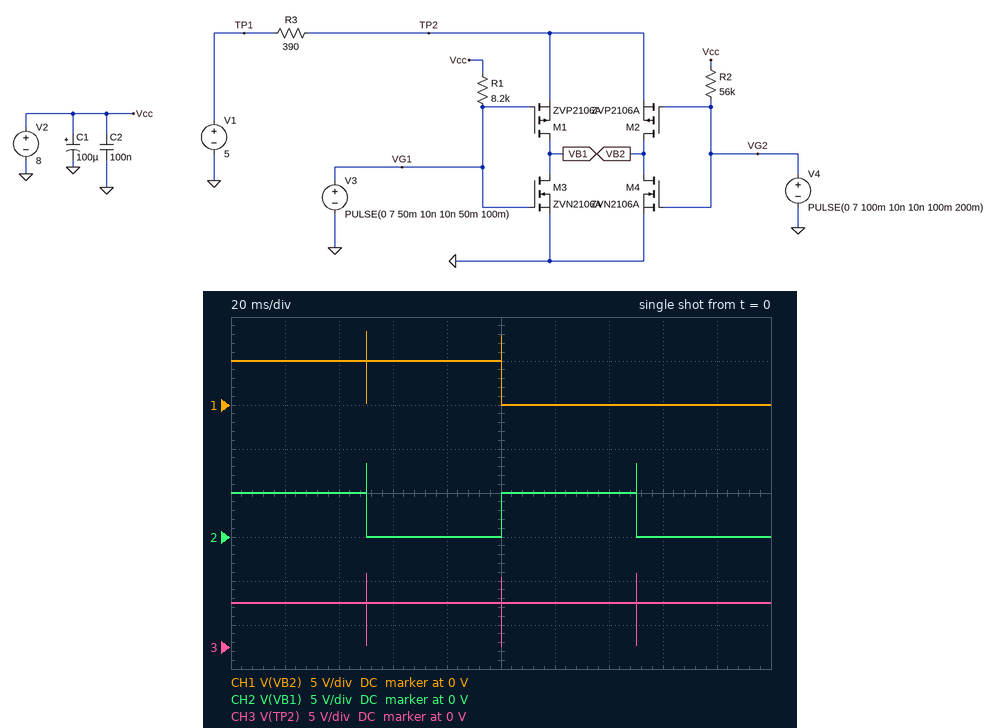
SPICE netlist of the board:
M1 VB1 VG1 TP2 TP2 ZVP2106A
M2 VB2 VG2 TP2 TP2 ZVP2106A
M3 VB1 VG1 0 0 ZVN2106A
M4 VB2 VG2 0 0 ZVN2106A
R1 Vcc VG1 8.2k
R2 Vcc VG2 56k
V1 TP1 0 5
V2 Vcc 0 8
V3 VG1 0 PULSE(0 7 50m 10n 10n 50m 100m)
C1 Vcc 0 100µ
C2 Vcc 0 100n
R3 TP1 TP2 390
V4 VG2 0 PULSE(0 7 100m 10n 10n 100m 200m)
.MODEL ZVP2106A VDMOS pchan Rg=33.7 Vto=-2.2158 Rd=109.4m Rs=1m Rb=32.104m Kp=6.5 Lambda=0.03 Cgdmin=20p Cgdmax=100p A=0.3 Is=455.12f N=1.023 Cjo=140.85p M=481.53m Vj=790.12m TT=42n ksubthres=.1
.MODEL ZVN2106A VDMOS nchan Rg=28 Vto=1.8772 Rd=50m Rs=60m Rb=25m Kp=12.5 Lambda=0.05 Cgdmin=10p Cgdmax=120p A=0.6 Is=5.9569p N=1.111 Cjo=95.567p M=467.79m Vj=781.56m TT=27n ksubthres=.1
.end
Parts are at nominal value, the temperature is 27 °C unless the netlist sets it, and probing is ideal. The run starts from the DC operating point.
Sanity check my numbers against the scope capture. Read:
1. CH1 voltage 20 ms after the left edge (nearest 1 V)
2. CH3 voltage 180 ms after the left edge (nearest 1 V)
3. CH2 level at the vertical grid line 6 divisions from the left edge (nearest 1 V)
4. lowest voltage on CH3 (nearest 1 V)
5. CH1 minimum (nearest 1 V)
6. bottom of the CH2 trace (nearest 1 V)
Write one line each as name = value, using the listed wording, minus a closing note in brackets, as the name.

CH1 voltage 20 ms after the left edge = 5 V
CH3 voltage 180 ms after the left edge = 5 V
CH2 level at the vertical grid line 6 divisions from the left edge = 5 V
lowest voltage on CH3 = 0 V
CH1 minimum = 0 V
bottom of the CH2 trace = 0 V
